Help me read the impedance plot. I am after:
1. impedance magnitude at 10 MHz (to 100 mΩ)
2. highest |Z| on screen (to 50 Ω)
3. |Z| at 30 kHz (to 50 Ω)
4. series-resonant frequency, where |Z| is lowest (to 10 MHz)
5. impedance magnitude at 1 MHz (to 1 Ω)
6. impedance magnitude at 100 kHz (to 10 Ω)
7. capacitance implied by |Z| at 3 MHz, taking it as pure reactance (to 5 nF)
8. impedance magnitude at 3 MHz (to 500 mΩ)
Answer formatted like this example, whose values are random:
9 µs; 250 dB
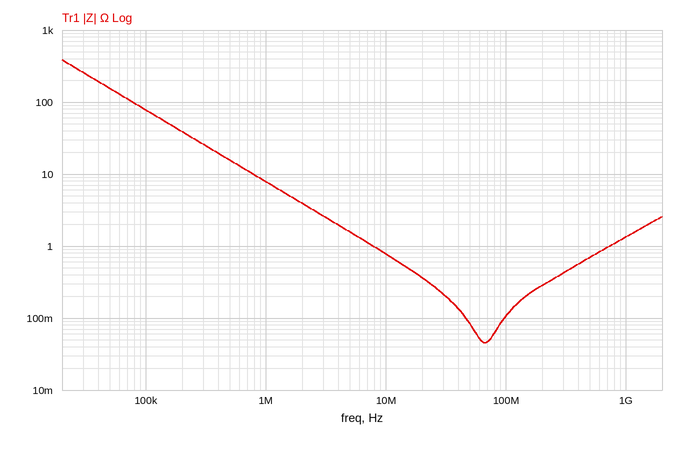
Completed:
800 mΩ; 400 Ω; 250 Ω; 70 MHz; 8 Ω; 80 Ω; 20 nF; 2.5 Ω
